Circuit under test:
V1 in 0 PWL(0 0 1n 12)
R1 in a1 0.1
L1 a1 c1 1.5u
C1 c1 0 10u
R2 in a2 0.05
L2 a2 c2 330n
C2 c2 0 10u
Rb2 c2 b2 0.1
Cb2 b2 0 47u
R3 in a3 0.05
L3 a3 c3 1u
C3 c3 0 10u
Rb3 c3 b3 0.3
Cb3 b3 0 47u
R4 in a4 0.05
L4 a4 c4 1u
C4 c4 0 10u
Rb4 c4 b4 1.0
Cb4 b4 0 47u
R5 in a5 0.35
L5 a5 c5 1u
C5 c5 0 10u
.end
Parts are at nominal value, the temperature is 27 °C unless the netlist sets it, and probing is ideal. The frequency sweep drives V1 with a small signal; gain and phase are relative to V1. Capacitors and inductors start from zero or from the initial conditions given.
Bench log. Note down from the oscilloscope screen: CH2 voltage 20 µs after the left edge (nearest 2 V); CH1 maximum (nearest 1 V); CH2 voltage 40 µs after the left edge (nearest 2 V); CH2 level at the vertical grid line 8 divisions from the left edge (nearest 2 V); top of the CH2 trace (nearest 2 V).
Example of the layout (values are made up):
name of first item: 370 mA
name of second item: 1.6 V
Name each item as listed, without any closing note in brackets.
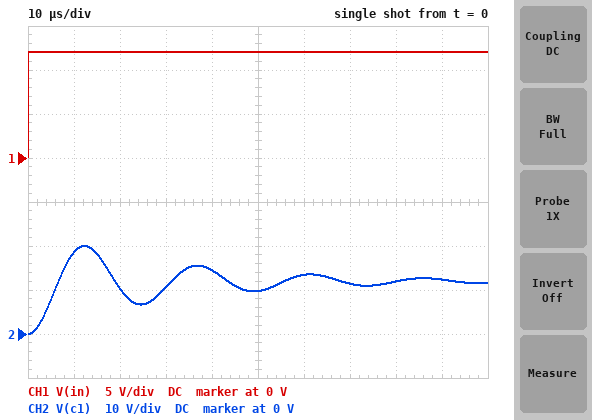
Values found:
CH2 voltage 20 µs after the left edge: 10 V
CH1 maximum: 12 V
CH2 voltage 40 µs after the left edge: 14 V
CH2 level at the vertical grid line 8 divisions from the left edge: 12 V
top of the CH2 trace: 20 V
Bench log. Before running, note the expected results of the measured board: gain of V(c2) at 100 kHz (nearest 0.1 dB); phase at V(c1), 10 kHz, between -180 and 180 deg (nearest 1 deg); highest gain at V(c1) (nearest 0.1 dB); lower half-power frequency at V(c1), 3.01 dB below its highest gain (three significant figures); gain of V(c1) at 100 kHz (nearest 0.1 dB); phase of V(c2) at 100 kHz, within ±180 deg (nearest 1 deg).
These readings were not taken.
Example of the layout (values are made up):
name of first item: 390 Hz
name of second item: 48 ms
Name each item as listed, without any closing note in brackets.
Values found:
gain of V(c2) at 100 kHz: -7.5 dB
phase at V(c1), 10 kHz, between -180 and 180 deg: -4 deg
highest gain at V(c1): 11.8 dB
lower half-power frequency at V(c1), 3.01 dB below its highest gain: 34.6 kHz
gain of V(c1) at 100 kHz: -13.9 dB
phase of V(c2) at 100 kHz, within ±180 deg: -102 deg
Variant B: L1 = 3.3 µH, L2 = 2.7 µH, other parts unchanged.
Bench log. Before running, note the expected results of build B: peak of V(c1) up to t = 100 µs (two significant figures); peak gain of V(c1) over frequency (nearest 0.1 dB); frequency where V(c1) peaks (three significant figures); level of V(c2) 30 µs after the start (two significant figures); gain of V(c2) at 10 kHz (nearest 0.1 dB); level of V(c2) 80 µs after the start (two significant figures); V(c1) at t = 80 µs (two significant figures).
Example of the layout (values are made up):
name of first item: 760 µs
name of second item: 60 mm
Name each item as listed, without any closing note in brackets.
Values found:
peak of V(c1) up to t = 100 µs: 21 V
peak gain of V(c1) over frequency: 15.2 dB
frequency where V(c1) peaks: 27.5 kHz
level of V(c2) 30 µs after the start: 17 V
gain of V(c2) at 10 kHz: 5.0 dB
level of V(c2) 80 µs after the start: 9.9 V
V(c1) at t = 80 µs: 11 V
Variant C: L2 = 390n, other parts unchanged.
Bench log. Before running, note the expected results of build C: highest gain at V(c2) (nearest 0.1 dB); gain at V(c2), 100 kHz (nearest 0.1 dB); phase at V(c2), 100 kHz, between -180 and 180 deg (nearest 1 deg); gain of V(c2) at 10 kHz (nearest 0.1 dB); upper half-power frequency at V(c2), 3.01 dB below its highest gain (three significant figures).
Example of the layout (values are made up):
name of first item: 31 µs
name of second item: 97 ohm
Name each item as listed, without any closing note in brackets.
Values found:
highest gain at V(c2): 0.5 dB
gain at V(c2), 100 kHz: -8.9 dB
phase at V(c2), 100 kHz, between -180 and 180 deg: -107 deg
gain of V(c2) at 10 kHz: 0.2 dB
upper half-power frequency at V(c2), 3.01 dB below its highest gain: 52.1 kHz
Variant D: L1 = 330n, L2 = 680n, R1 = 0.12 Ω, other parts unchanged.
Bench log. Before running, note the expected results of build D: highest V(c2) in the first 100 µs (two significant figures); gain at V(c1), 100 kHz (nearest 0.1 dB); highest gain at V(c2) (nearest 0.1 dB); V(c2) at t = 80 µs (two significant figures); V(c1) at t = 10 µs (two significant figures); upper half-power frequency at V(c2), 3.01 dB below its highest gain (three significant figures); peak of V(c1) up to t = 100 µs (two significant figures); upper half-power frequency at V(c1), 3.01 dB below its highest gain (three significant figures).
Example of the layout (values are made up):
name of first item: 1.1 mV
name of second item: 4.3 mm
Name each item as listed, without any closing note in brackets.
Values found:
highest V(c2) in the first 100 µs: 14 V
gain at V(c1), 100 kHz: 1.8 dB
highest gain at V(c2): 1.7 dB
V(c2) at t = 80 µs: 12 V
V(c1) at t = 10 µs: 12 V
upper half-power frequency at V(c2), 3.01 dB below its highest gain: 35.3 kHz
peak of V(c1) up to t = 100 µs: 16 V
upper half-power frequency at V(c1), 3.01 dB below its highest gain: 104 kHz
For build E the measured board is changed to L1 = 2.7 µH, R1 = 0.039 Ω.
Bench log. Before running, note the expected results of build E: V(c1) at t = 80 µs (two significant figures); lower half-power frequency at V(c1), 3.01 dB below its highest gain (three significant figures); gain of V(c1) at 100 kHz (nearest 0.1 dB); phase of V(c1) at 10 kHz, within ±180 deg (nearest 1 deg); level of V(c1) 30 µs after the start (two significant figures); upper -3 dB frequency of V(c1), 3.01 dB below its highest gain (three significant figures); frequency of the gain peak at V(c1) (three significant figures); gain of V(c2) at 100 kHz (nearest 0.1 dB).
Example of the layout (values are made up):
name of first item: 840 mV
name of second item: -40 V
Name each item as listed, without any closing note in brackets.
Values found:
V(c1) at t = 80 µs: 18 V
lower half-power frequency at V(c1), 3.01 dB below its highest gain: 29.4 kHz
gain of V(c1) at 100 kHz: -19.7 dB
phase of V(c1) at 10 kHz, within ±180 deg: -2 deg
level of V(c1) 30 µs after the start: 3.8 V
upper -3 dB frequency of V(c1), 3.01 dB below its highest gain: 31.7 kHz
frequency of the gain peak at V(c1): 30.6 kHz
gain of V(c2) at 100 kHz: -7.5 dB
